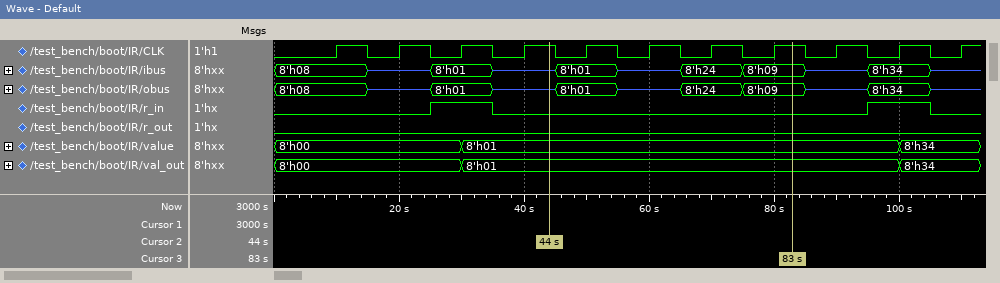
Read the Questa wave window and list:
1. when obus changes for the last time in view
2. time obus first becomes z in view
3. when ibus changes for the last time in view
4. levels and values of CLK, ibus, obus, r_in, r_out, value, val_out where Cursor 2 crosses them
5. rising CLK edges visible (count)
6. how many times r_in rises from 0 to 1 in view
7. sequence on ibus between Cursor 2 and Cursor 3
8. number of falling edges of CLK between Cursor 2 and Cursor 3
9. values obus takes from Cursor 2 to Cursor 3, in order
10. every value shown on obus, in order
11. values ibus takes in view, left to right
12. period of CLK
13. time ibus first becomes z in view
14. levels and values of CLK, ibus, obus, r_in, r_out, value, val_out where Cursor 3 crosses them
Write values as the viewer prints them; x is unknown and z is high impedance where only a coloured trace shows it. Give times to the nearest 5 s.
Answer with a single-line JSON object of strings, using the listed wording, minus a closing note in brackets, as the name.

{"when obus changes for the last time in view": "105 s", "time obus first becomes z in view": "15 s", "when ibus changes for the last time in view": "105 s", "levels and values of CLK, ibus, obus, r_in, r_out, value, val_out where Cursor 2 crosses them": "CLK=1, ibus=z, obus=z, r_in=0, r_out=0, value=8'h01, val_out=8'h01", "rising CLK edges visible": "11", "how many times r_in rises from 0 to 1 in view": "2", "sequence on ibus between Cursor 2 and Cursor 3": "z, 8'h01, z, 8'h24, 8'h09", "number of falling edges of CLK between Cursor 2 and Cursor 3": "4", "values obus takes from Cursor 2 to Cursor 3, in order": "z, 8'h01, z, 8'h24, 8'h09", "every value shown on obus, in order": "8'h08, z, 8'h01, z, 8'h01, z, 8'h24, 8'h09, z, 8'h34, z", "values ibus takes in view, left to right": "8'h08, z, 8'h01, z, 8'h01, z, 8'h24, 8'h09, z, 8'h34, z", "period of CLK": "10 s", "time ibus first becomes z in view": "15 s", "levels and values of CLK, ibus, obus, r_in, r_out, value, val_out where Cursor 3 crosses them": "CLK=1, ibus=8'h09, obus=8'h09, r_in=0, r_out=0, value=8'h01, val_out=8'h01"}
